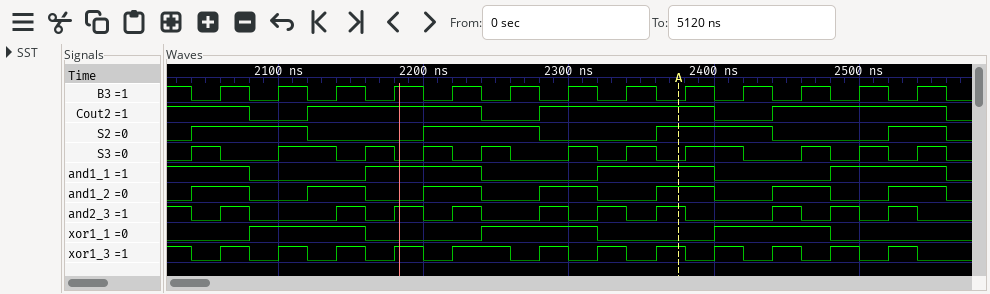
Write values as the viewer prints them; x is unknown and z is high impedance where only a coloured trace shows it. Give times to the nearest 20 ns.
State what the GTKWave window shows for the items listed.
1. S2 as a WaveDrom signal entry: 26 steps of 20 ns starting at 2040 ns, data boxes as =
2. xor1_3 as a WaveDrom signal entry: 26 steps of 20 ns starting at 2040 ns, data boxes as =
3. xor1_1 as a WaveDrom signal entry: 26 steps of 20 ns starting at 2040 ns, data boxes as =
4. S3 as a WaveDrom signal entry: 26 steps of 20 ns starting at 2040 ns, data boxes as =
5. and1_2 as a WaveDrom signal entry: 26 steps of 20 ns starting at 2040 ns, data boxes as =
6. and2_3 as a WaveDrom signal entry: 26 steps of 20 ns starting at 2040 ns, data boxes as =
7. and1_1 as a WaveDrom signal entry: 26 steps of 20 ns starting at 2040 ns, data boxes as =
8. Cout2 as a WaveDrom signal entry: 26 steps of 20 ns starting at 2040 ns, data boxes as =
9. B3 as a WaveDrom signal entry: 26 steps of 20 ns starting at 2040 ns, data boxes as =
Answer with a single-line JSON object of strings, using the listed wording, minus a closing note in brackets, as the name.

{"S2 as a WaveDrom signal entry: 26 steps of 20 ns starting at 2040 ns, data boxes as =": "{name: 'S2', wave: '1...0...1...0...1...0...1.'}", "xor1_3 as a WaveDrom signal entry: 26 steps of 20 ns starting at 2040 ns, data boxes as =": "{name: 'xor1_3', wave: '0101010101.010101010101010'}", "xor1_1 as a WaveDrom signal entry: 26 steps of 20 ns starting at 2040 ns, data boxes as =": "{name: 'xor1_1', wave: '0.1...0...1...0...1...0...'}", "S3 as a WaveDrom signal entry: 26 steps of 20 ns starting at 2040 ns, data boxes as =": "{name: 'S3', wave: '10.1.0101010.10101.0.10101'}", "and1_2 as a WaveDrom signal entry: 26 steps of 20 ns starting at 2040 ns, data boxes as =": "{name: 'and1_2', wave: '1.0.1.0.1.0.1.0.1.0.1.0.1.'}", "and2_3 as a WaveDrom signal entry: 26 steps of 20 ns starting at 2040 ns, data boxes as =": "{name: 'and2_3', wave: '010..101010.101010..101010'}", "and1_1 as a WaveDrom signal entry: 26 steps of 20 ns starting at 2040 ns, data boxes as =": "{name: 'and1_1', wave: '1.0...1...0...1...0...1...'}", "Cout2 as a WaveDrom signal entry: 26 steps of 20 ns starting at 2040 ns, data boxes as =": "{name: 'Cout2', wave: '1.0.1.....0.1.....0.1.....'}", "B3 as a WaveDrom signal entry: 26 steps of 20 ns starting at 2040 ns, data boxes as =": "{name: 'B3', wave: '01010101010101010101010101'}"}
